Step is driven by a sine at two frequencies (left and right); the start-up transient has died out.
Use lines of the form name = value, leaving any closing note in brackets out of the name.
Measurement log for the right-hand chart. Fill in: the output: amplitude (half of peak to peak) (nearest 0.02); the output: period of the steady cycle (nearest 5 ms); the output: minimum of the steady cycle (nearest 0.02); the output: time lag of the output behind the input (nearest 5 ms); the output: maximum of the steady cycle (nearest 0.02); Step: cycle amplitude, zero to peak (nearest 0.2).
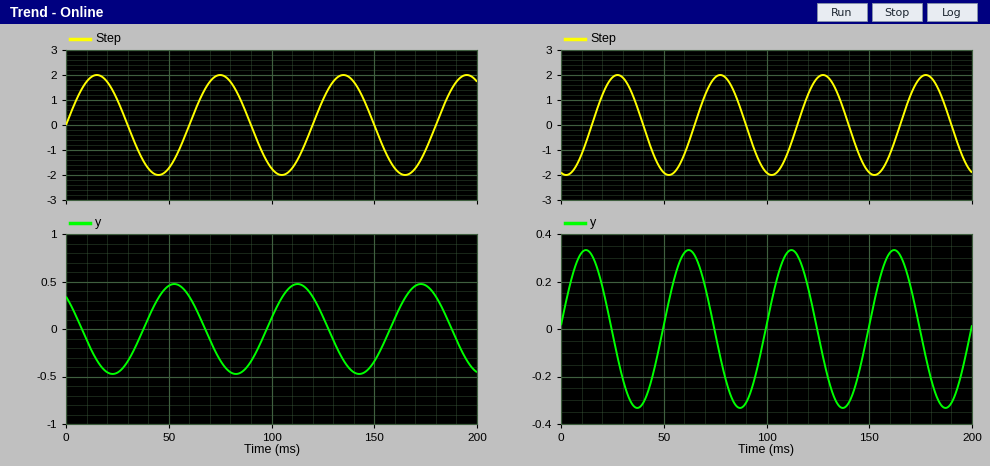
the output: amplitude (half of peak to peak) = 0.34
the output: period of the steady cycle = 50 ms
the output: minimum of the steady cycle = -0.34
the output: time lag of the output behind the input = 35 ms
the output: maximum of the steady cycle = 0.34
Step: cycle amplitude, zero to peak = 2.0
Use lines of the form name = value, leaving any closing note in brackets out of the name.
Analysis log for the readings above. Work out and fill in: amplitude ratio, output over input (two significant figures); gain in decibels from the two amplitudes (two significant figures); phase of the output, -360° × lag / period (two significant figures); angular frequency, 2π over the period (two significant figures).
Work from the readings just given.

amplitude ratio, output over input = 0.17
gain in decibels from the two amplitudes = -15 dB
phase of the output, -360° × lag / period = -250°
angular frequency, 2π over the period = 0.13 rad/ms
